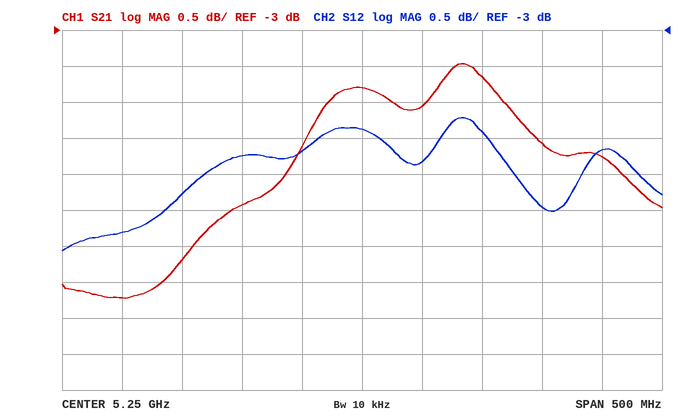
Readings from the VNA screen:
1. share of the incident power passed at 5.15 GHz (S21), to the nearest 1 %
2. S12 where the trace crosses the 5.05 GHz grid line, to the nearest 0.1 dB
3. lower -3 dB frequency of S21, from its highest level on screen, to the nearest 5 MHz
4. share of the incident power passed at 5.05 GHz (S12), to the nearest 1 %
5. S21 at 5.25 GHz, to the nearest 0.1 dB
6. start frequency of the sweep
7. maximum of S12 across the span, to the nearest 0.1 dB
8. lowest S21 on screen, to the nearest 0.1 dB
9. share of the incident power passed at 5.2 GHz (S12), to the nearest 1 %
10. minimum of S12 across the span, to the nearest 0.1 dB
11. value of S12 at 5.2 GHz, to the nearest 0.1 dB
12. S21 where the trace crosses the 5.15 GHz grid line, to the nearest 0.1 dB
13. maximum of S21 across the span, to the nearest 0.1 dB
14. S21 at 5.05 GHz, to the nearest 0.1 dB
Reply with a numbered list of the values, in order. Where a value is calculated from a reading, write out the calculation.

1. 10^(-5.4/10) ≈ 29 %
2. -5.8 dB
3. 5.085 GHz
4. 10^(-5.8/10) ≈ 26 %
5. -3.8 dB
6. 5 GHz
7. -4.2 dB
8. -6.7 dB
9. 10^(-4.7/10) ≈ 34 %
10. -6.1 dB
11. -4.7 dB
12. -5.4 dB
13. -3.5 dB
14. -6.7 dB
